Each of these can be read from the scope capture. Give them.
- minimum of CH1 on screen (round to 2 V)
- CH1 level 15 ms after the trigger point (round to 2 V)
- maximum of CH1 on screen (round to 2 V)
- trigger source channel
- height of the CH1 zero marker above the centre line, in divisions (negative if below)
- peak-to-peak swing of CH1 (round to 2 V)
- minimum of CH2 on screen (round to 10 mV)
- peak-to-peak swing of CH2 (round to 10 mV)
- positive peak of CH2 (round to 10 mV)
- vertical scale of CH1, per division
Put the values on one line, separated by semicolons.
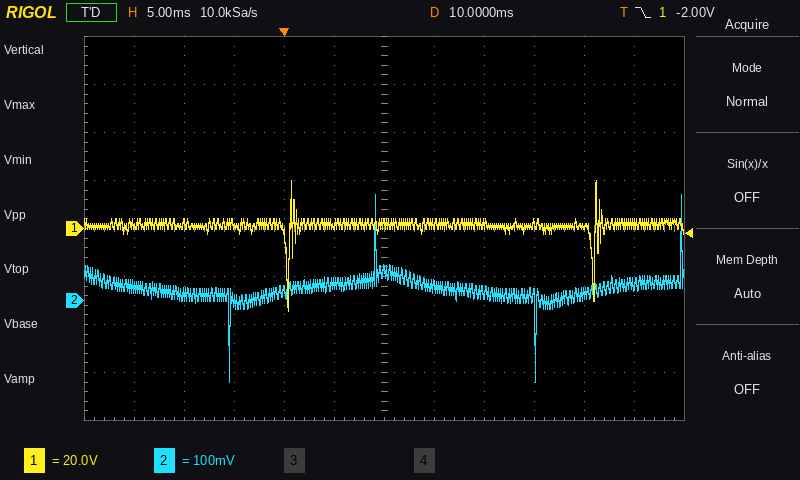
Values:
-34 V; 2 V; 20 V; CH1; 0.0 div; 54 V; -170 mV; 390 mV; 220 mV; 20 V
